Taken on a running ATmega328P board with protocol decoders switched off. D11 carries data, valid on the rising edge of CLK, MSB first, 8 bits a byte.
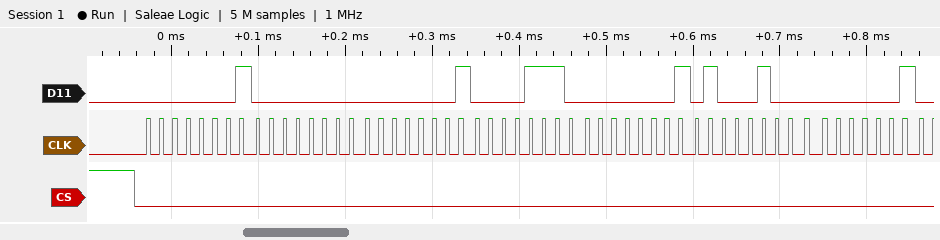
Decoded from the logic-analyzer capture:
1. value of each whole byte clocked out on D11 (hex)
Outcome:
01 00 01 0E 01 44 01
